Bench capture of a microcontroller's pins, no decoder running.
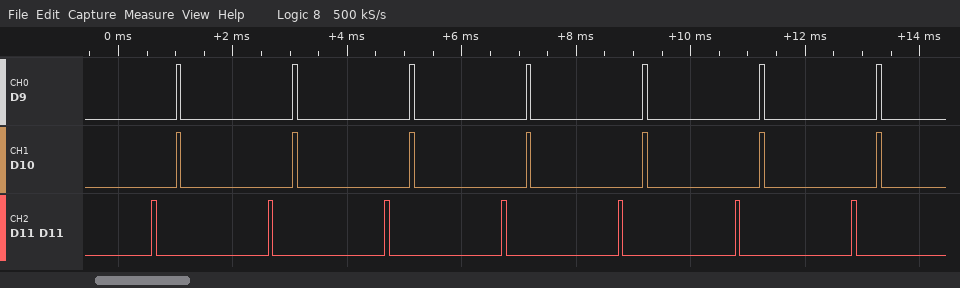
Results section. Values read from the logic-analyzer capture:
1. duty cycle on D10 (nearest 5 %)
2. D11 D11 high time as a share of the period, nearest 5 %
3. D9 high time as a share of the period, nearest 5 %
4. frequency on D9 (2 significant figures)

5 %
5 %
5 %
490 Hz
